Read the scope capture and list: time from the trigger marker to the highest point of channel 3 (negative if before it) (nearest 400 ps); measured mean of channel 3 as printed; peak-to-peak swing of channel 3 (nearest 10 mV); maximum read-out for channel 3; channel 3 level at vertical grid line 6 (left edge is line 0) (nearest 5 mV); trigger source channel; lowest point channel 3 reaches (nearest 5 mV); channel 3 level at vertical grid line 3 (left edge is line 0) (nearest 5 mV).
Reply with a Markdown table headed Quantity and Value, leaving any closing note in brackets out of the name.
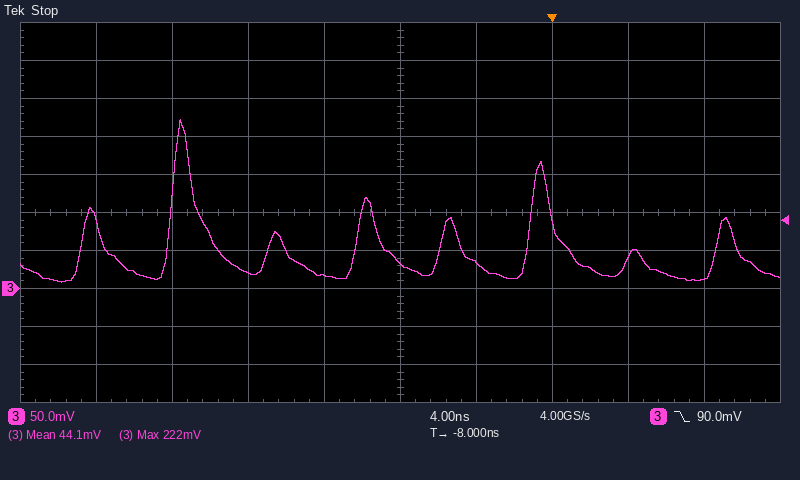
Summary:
| Quantity | Value |
|---|---|
| time from the trigger marker to the highest point of channel 3 (negative if before it) | -19.6 ns |
| measured mean of channel 3 as printed | 44.1 mV |
| peak-to-peak swing of channel 3 | 210 mV |
| maximum read-out for channel 3 | 222 mV |
| channel 3 level at vertical grid line 6 (left edge is line 0) | 35 mV |
| trigger source channel | channel 3 |
| lowest point channel 3 reaches | 10 mV |
| channel 3 level at vertical grid line 3 (left edge is line 0) | 20 mV |
